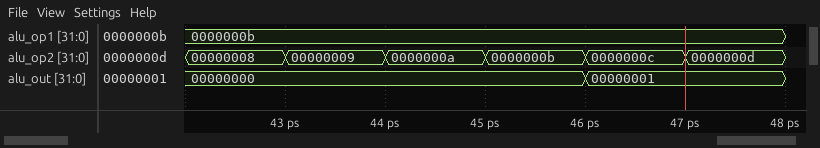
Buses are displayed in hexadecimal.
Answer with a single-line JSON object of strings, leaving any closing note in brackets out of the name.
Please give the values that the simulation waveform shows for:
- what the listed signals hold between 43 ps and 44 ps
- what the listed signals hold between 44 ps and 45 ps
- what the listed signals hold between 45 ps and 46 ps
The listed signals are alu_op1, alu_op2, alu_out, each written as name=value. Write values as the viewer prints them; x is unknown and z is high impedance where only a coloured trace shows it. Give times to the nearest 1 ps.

{"what the listed signals hold between 43 ps and 44 ps": "alu_op1=0000000b, alu_op2=00000009, alu_out=00000000", "what the listed signals hold between 44 ps and 45 ps": "alu_op1=0000000b, alu_op2=0000000a, alu_out=00000000", "what the listed signals hold between 45 ps and 46 ps": "alu_op1=0000000b, alu_op2=0000000b, alu_out=00000000"}
